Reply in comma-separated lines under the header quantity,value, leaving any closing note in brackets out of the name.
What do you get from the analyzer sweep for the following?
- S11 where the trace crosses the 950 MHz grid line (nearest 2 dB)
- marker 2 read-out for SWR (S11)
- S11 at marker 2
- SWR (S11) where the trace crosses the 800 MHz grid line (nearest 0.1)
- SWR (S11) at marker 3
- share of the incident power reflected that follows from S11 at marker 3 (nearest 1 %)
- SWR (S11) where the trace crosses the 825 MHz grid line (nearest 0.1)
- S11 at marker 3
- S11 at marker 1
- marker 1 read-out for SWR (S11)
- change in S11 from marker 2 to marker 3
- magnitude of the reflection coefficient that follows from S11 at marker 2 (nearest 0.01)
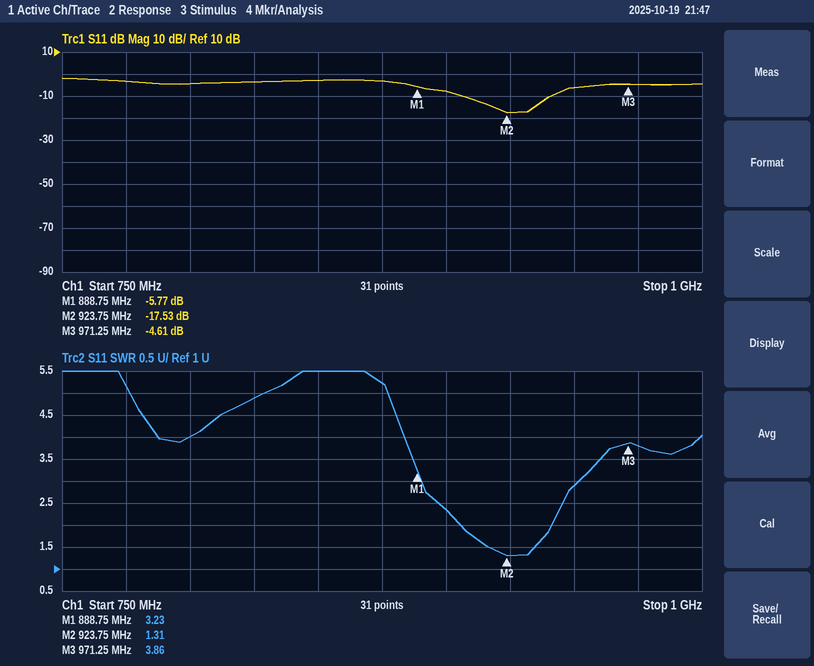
quantity,value
S11 where the trace crosses the 950 MHz grid line,-6 dB
marker 2 read-out for SWR,1.31
S11 at marker 2,-17.53 dB
SWR (S11) where the trace crosses the 800 MHz grid line,4.0
SWR (S11) at marker 3,3.86
share of the incident power reflected that follows from S11 at marker 3,35 %
SWR (S11) where the trace crosses the 825 MHz grid line,4.9
S11 at marker 3,-4.61 dB
S11 at marker 1,-5.77 dB
marker 1 read-out for SWR,3.23
change in S11 from marker 2 to marker 3,12.92 dB
magnitude of the reflection coefficient that follows from S11 at marker 2,0.13
